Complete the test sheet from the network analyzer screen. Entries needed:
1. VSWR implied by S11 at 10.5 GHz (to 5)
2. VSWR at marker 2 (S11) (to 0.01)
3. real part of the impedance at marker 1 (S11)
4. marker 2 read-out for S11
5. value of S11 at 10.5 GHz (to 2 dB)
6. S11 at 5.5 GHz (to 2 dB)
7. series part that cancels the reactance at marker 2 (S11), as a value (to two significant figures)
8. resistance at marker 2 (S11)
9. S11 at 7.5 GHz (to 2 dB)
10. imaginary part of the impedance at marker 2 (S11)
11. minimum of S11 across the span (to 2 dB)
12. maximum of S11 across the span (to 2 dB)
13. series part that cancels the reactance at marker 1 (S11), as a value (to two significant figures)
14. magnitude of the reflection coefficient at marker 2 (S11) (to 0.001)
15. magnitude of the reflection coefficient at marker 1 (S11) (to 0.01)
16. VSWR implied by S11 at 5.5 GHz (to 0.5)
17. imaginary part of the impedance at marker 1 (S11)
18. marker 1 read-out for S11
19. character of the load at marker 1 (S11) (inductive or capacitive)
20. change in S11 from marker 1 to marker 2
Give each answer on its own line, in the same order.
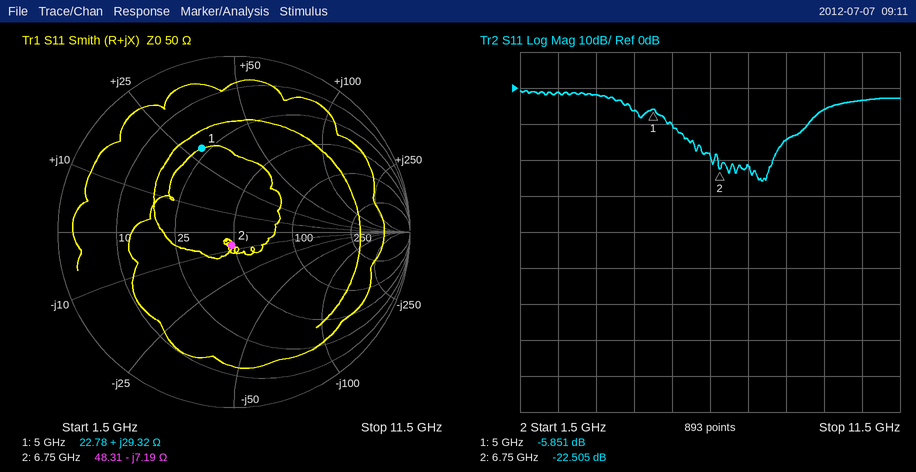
5
1.16
22.78 Ω
-22.505 dB
-4 dB
-10 dB
170 pH
48.31 Ω
-22 dB
-7.19 Ω
-26 dB
0 dB
1.1 pF
0.075
0.51
2.0
+29.32 Ω
-5.851 dB
inductive
-16.654 dB
